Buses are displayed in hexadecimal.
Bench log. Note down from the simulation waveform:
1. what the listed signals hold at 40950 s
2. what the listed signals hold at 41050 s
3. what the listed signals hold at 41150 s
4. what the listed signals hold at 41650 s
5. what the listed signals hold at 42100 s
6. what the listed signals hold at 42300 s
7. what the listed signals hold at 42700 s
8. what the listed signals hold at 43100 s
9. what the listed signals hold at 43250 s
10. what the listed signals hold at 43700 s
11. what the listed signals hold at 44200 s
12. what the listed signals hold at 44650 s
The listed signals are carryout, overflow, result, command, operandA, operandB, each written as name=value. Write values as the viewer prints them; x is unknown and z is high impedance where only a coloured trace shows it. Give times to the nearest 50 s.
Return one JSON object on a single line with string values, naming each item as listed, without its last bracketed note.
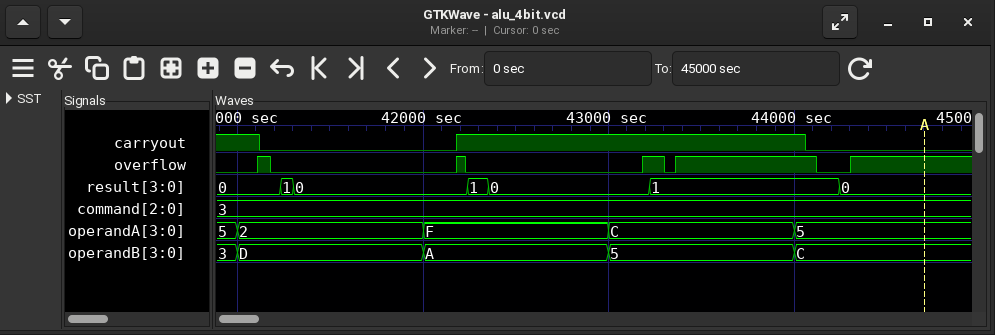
{"what the listed signals hold at 40950 s": "carryout=1, overflow=0, result=0, command=3, operandA=5, operandB=3", "what the listed signals hold at 41050 s": "carryout=1, overflow=0, result=0, command=3, operandA=2, operandB=D", "what the listed signals hold at 41150 s": "carryout=0, overflow=1, result=0, command=3, operandA=2, operandB=D", "what the listed signals hold at 41650 s": "carryout=0, overflow=0, result=0, command=3, operandA=2, operandB=D", "what the listed signals hold at 42100 s": "carryout=0, overflow=0, result=0, command=3, operandA=F, operandB=A", "what the listed signals hold at 42300 s": "carryout=1, overflow=0, result=1, command=3, operandA=F, operandB=A", "what the listed signals hold at 42700 s": "carryout=1, overflow=0, result=0, command=3, operandA=F, operandB=A", "what the listed signals hold at 43100 s": "carryout=1, overflow=0, result=0, command=3, operandA=C, operandB=5", "what the listed signals hold at 43250 s": "carryout=1, overflow=1, result=1, command=3, operandA=C, operandB=5", "what the listed signals hold at 43700 s": "carryout=1, overflow=1, result=1, command=3, operandA=C, operandB=5", "what the listed signals hold at 44200 s": "carryout=0, overflow=0, result=1, command=3, operandA=5, operandB=C", "what the listed signals hold at 44650 s": "carryout=0, overflow=1, result=0, command=3, operandA=5, operandB=C"}
